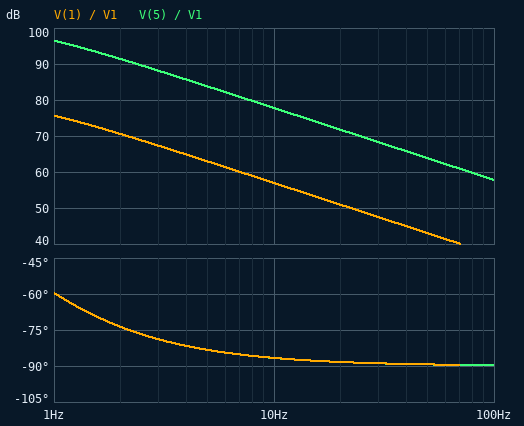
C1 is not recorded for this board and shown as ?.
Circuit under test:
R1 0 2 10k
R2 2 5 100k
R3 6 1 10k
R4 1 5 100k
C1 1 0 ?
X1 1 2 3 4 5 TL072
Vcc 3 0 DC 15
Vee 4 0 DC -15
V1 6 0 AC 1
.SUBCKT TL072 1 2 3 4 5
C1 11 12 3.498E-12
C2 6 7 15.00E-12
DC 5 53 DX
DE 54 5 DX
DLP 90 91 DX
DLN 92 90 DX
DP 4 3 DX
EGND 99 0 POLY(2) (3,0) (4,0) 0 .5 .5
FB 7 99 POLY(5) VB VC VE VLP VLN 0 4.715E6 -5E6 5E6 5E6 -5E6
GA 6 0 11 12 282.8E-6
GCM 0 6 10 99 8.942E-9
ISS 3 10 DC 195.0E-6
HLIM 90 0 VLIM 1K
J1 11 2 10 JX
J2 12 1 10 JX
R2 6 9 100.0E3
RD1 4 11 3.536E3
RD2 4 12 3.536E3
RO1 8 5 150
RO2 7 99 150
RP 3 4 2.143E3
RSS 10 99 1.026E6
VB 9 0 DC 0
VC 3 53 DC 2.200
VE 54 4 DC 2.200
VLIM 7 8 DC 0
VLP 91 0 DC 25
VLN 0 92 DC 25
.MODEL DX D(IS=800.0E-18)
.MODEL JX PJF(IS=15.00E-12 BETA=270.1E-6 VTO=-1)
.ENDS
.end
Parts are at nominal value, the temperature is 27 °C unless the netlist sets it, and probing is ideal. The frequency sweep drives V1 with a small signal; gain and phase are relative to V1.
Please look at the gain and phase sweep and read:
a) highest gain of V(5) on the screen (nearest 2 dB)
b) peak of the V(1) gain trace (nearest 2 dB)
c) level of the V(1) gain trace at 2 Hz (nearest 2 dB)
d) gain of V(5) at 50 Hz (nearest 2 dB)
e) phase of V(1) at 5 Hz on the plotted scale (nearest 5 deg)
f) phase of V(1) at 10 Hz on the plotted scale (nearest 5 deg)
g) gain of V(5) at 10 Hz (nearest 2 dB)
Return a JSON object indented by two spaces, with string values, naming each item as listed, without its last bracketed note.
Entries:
{
  "highest gain of V(5) on the screen": "96 dB",
  "peak of the V(1) gain trace": "76 dB",
  "level of the V(1) gain trace at 2 Hz": "70 dB",
  "gain of V(5) at 50 Hz": "64 dB",
  "phase of V(1) at 5 Hz on the plotted scale": "-85 deg",
  "phase of V(1) at 10 Hz on the plotted scale": "-85 deg",
  "gain of V(5) at 10 Hz": "78 dB"
}
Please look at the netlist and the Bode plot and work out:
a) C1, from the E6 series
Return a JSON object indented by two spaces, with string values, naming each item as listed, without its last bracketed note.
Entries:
{
  "C1, from the E6 series": "2.2 nF"
}
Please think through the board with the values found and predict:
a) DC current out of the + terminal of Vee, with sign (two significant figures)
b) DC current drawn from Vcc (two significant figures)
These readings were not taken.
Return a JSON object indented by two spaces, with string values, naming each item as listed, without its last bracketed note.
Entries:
{
  "DC current out of the + terminal of Vee, with sign": "-14 mA",
  "DC current drawn from Vcc": "14 mA"
}
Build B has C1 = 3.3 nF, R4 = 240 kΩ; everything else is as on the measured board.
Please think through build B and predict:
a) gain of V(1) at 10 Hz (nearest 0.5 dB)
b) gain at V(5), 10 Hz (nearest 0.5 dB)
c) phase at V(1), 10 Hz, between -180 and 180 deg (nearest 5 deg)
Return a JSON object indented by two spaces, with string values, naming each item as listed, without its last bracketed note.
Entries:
{
  "gain of V(1) at 10 Hz": "4.5 dB",
  "gain at V(5), 10 Hz": "25.5 dB",
  "phase at V(1), 10 Hz, between -180 and 180 deg": "0 deg"
}
